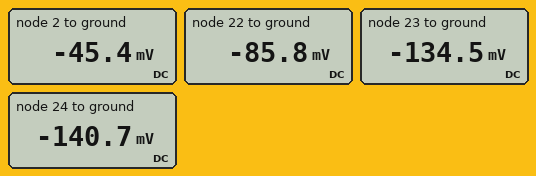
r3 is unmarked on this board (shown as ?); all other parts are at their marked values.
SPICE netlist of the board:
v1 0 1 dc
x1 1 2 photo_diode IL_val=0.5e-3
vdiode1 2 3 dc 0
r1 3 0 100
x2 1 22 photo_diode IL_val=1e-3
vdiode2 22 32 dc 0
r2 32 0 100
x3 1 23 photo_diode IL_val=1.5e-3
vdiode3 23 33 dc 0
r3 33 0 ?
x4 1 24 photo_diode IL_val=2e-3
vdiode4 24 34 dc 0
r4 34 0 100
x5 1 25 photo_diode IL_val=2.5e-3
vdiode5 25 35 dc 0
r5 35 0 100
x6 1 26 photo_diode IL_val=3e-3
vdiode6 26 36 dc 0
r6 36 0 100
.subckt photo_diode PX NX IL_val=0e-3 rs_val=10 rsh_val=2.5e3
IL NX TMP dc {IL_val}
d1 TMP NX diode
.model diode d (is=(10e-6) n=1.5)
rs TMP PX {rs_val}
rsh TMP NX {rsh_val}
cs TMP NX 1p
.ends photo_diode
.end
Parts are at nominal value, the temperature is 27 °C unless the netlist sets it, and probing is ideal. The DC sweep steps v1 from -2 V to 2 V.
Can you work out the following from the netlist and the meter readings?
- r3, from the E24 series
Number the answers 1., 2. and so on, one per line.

1. 130 Ω
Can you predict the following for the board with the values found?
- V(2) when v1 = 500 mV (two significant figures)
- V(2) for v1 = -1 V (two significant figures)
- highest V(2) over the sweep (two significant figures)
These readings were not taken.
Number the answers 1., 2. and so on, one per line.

1. -68 mV
2. 680 mV
3. 1.6 V
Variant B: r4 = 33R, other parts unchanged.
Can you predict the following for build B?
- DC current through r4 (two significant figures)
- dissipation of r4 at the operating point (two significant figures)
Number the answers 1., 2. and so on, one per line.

1. 1.9 mA
2. 120 µW
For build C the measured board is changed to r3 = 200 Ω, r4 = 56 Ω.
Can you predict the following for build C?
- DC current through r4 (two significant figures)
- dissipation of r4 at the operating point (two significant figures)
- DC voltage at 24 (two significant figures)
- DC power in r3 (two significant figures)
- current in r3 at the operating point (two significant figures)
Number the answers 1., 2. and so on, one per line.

1. 1.8 mA
2. 170 µW
3. -99 mV
4. 120 µW
5. 780 µA
